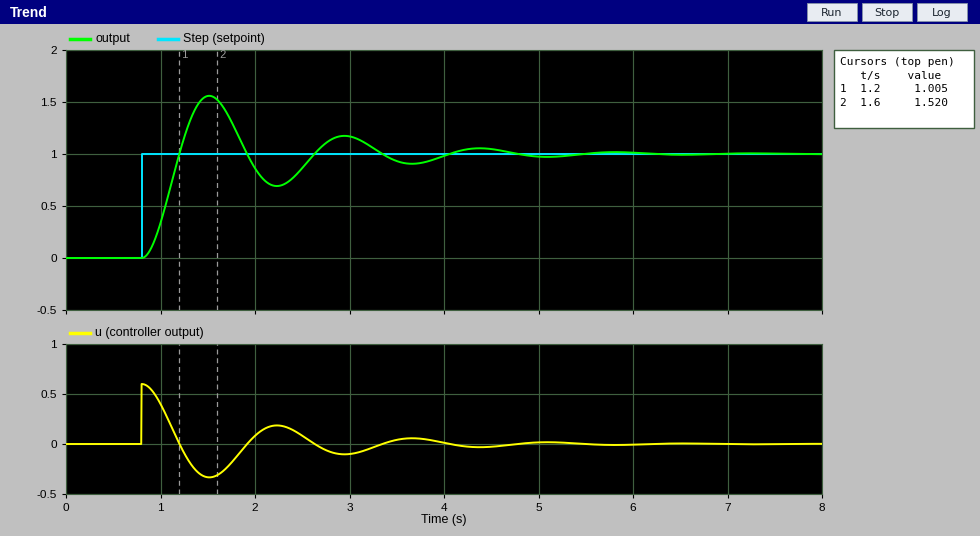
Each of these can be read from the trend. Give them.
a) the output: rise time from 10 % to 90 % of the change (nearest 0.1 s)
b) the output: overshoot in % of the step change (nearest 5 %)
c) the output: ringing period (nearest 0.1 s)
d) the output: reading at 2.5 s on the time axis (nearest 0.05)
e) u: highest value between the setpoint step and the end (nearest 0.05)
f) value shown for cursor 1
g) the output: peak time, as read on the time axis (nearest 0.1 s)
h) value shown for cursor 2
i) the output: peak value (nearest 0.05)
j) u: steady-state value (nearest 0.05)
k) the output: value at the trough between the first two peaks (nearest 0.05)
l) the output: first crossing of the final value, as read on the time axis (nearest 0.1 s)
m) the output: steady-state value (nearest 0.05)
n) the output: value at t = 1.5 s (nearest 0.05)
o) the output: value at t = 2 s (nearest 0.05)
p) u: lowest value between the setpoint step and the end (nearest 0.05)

0.3 s
55 %
1.4 s
0.85
0.60
1.005
1.5 s
1.520
1.55
0.00
0.70
1.2 s
1.00
1.55
0.85
-0.35
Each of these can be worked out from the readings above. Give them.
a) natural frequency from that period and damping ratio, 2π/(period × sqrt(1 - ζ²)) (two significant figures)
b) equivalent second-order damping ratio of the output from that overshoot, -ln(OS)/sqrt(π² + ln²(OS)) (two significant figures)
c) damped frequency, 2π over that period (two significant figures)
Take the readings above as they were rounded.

4.6 rad/s
0.19
4.5 rad/s
